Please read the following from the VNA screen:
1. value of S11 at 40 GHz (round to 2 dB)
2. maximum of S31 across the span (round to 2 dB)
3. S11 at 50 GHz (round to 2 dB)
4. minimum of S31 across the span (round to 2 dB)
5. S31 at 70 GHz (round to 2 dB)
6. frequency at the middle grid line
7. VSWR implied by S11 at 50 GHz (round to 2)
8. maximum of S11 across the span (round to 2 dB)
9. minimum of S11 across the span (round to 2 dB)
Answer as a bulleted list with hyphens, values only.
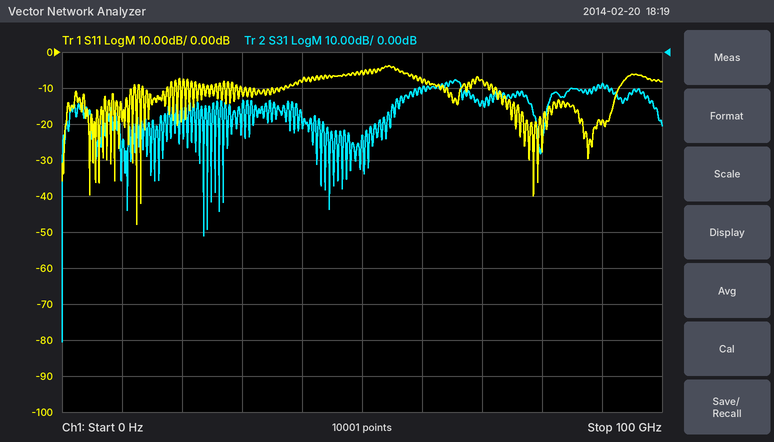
- -8 dB
- -8 dB
- -6 dB
- -80 dB
- -14 dB
- 50 GHz
- 4
- -4 dB
- -48 dB
